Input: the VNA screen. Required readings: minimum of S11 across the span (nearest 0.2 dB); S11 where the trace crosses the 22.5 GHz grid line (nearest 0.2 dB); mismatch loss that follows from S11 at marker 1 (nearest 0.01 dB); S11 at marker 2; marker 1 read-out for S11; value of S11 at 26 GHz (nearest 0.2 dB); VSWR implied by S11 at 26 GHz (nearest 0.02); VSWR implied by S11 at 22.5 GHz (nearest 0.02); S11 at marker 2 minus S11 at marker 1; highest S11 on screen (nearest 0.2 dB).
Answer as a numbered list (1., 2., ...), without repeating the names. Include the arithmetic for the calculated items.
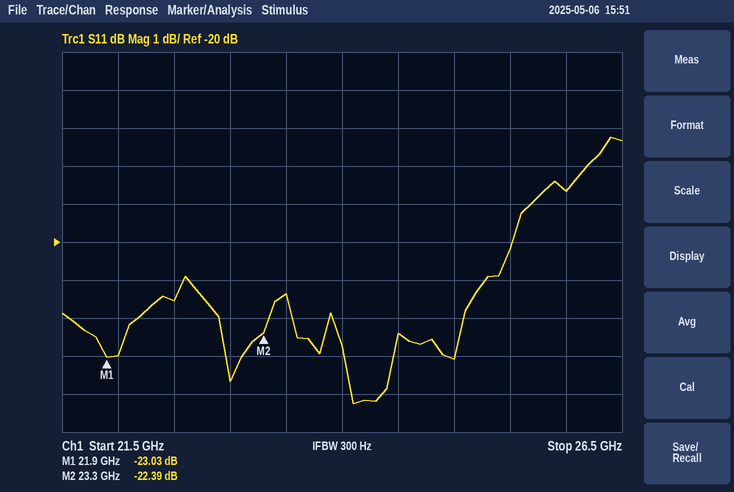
1. -24.2 dB
2. -21.6 dB
3. −10 log10(1 − 10^(-23.03/10)) ≈ 0.02 dB
4. -22.39 dB
5. -23.03 dB
6. -18.6 dB
7. |Γ| = 10^(-18.6/20) = 0.1175; VSWR = (1 + 0.1175)/(1 − 0.1175) ≈ 1.27, so 1.26 to the nearest 0.02
8. |Γ| = 10^(-21.6/20) = 0.0832; VSWR = (1 + 0.0832)/(1 − 0.0832) ≈ 1.18
9. -22.39 − (-23.03) = 0.64 dB
10. -17.2 dB
